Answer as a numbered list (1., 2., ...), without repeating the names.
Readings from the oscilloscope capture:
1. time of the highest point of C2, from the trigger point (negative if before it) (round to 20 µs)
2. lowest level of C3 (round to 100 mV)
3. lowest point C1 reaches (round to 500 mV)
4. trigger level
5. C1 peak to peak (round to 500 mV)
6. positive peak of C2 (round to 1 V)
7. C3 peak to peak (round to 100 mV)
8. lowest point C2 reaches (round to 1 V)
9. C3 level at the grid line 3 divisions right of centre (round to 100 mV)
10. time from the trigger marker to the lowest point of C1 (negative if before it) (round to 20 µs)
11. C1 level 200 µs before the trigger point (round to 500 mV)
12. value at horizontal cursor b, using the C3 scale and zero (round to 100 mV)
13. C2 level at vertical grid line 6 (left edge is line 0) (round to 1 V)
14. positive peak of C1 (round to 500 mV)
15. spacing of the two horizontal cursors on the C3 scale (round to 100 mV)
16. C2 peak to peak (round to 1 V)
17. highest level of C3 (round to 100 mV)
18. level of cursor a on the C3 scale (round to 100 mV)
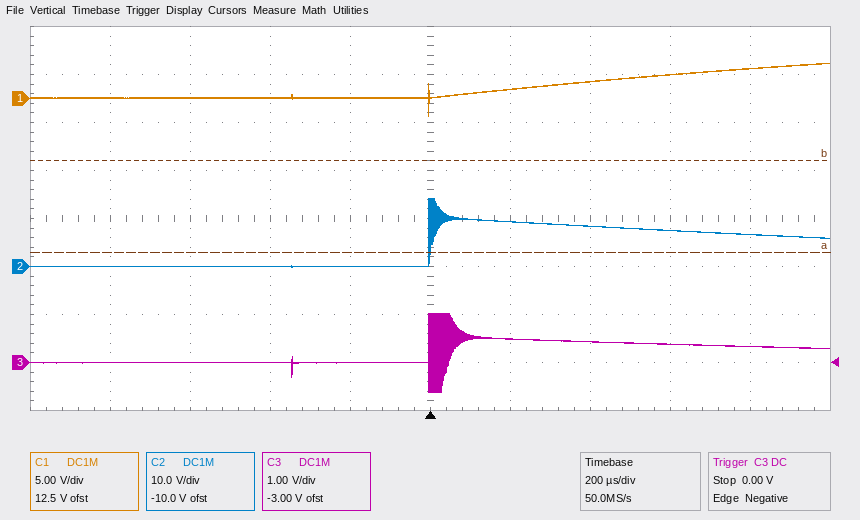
1. 0 µs
2. -600 mV
3. -2.0 V
4. 0.00 V
5. 5.5 V
6. 14 V
7. 1.6 V
8. 0 V
9. 400 mV
10. 0 µs
11. 0.0 V
12. 4.2 V
13. 9 V
14. 3.5 V
15. 1.9 V
16. 14 V
17. 1.0 V
18. 2.3 V
